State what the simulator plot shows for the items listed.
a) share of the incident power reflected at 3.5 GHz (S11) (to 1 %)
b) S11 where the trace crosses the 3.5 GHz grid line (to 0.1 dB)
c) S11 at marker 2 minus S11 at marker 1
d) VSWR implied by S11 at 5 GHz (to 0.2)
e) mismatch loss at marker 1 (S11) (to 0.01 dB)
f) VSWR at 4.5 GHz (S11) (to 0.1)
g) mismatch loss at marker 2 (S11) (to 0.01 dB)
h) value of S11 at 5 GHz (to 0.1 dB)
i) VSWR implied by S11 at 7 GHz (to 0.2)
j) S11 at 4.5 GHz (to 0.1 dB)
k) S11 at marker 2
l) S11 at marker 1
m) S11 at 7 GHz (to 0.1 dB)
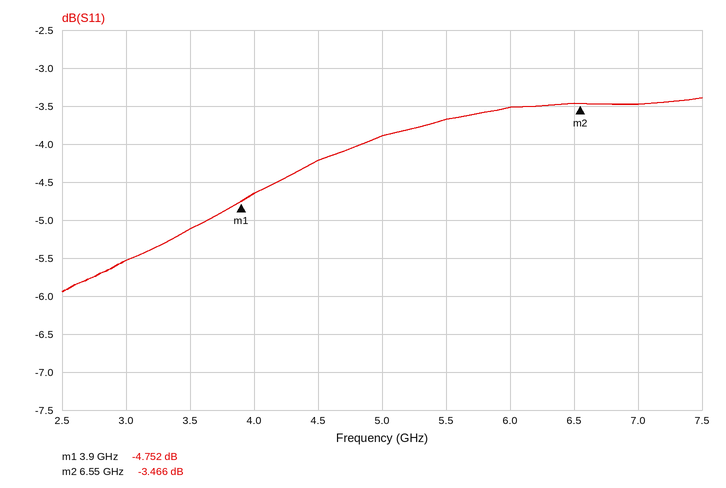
31 %
-5.1 dB
1.286 dB
4.6
1.77 dB
4.2
2.60 dB
-3.9 dB
5.0
-4.2 dB
-3.466 dB
-4.752 dB
-3.5 dB
